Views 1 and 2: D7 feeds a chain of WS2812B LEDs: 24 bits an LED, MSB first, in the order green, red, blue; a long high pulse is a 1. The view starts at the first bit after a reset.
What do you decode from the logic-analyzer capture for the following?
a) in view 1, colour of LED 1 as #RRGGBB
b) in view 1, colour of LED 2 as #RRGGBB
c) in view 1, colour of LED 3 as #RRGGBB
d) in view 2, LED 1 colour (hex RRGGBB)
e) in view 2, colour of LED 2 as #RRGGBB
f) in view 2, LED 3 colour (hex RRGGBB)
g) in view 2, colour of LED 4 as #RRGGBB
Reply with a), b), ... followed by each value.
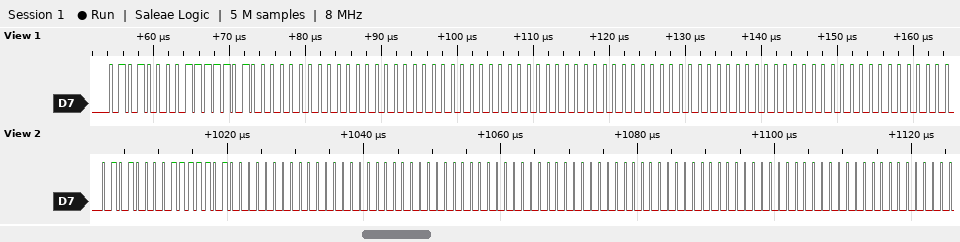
a) #FA5000
b) #000000
c) #000000
d) #FA5000
e) #000000
f) #000000
g) #000000
